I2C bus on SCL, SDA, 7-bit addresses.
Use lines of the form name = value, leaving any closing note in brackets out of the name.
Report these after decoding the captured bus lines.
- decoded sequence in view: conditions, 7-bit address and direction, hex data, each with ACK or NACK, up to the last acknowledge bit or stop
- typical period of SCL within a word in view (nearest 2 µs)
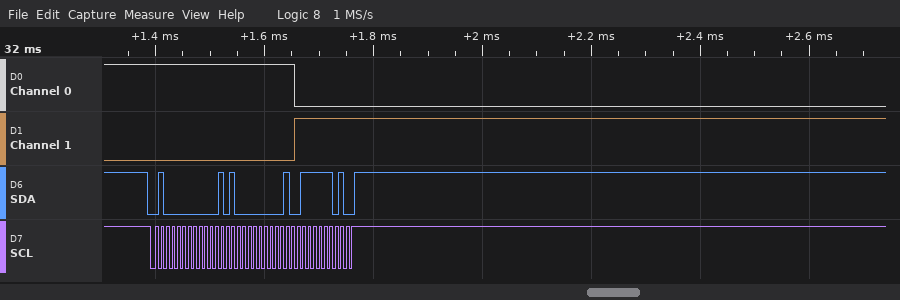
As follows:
decoded sequence in view: conditions, 7-bit address and direction, hex data, each with ACK or NACK, up to the last acknowledge bit or stop = start, address 20 write ACK, 14 ACK, 02 ACK, FD ACK, stop
typical period of SCL within a word in view = 10 µs
